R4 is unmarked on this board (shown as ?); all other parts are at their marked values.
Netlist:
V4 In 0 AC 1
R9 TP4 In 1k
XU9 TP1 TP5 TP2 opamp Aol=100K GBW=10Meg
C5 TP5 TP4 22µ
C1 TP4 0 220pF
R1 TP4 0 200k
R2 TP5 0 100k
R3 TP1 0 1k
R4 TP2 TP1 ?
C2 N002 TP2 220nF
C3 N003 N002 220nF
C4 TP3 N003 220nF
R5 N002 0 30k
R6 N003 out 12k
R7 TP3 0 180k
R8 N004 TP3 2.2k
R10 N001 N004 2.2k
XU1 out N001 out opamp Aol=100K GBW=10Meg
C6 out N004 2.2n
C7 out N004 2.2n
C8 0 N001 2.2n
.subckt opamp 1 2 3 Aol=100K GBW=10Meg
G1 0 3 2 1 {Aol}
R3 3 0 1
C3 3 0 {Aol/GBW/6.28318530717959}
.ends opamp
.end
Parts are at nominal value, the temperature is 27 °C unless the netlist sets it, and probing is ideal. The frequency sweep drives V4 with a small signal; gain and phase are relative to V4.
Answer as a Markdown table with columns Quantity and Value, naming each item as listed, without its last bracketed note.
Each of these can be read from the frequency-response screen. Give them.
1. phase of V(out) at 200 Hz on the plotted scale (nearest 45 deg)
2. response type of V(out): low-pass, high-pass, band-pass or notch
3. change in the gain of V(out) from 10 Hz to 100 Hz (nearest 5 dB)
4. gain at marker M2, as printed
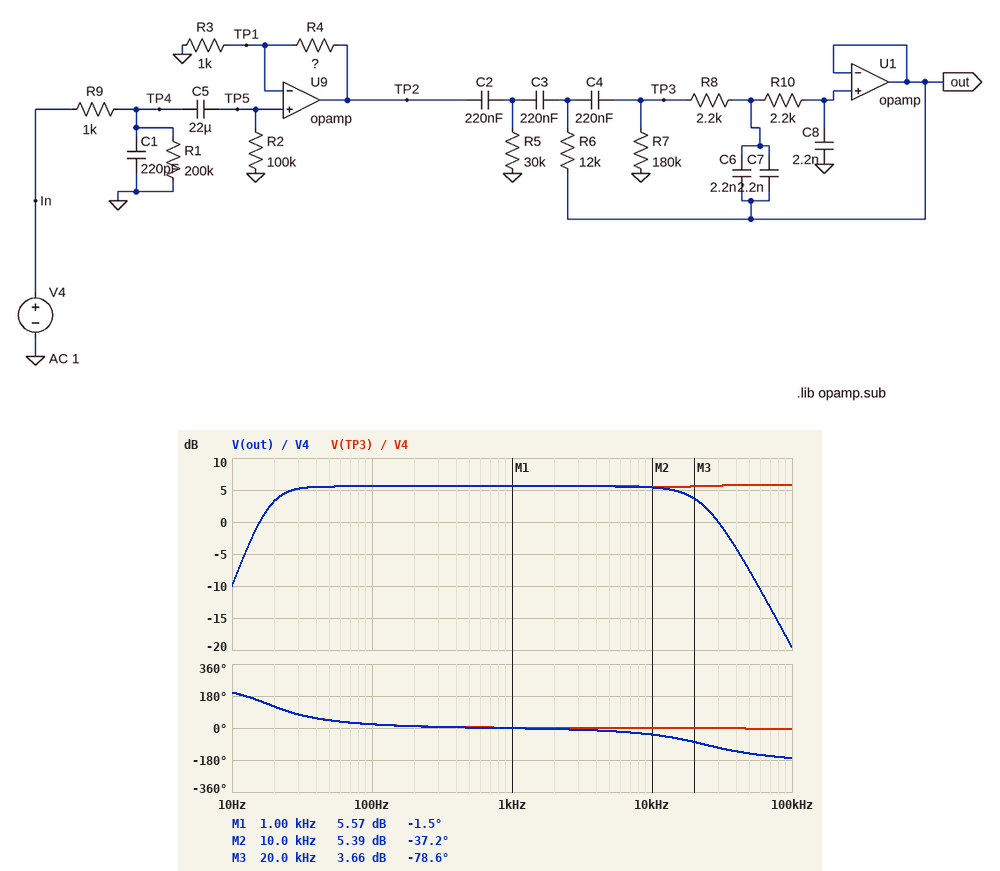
| Quantity | Value |
|---|---|
| phase of V(out) at 200 Hz on the plotted scale | 0 deg |
| response type of V(out): low-pass, high-pass, band-pass or notch | band-pass |
| change in the gain of V(out) from 10 Hz to 100 Hz | 15 dB |
| gain at marker M2, as printed | 5.39 dB |
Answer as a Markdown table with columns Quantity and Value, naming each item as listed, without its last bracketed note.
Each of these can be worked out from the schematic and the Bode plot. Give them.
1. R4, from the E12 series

| Quantity | Value |
|---|---|
| R4, from the E12 series | 1 kΩ |
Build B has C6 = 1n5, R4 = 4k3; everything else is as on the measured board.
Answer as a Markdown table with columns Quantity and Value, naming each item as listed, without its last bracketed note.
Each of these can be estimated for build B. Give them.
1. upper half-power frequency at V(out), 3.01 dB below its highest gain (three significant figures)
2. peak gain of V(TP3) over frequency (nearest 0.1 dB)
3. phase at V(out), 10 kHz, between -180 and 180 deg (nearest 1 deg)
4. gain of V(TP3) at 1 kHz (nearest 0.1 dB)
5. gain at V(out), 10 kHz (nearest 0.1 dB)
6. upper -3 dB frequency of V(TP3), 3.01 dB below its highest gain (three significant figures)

| Quantity | Value |
|---|---|
| upper half-power frequency at V(out), 3.01 dB below its highest gain | 23.2 kHz |
| peak gain of V(TP3) over frequency | 14.3 dB |
| phase at V(out), 10 kHz, between -180 and 180 deg | -36 deg |
| gain of V(TP3) at 1 kHz | 14.0 dB |
| gain at V(out), 10 kHz | 13.7 dB |
| upper -3 dB frequency of V(TP3), 3.01 dB below its highest gain | 663 kHz |
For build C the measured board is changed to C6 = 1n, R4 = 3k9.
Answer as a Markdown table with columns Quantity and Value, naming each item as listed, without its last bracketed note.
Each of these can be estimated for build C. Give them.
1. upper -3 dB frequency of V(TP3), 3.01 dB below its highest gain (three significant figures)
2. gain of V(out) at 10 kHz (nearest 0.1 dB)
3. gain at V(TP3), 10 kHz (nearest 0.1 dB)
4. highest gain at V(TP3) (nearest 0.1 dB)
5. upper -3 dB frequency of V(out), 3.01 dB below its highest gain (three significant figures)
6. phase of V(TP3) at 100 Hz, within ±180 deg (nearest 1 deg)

| Quantity | Value |
|---|---|
| upper -3 dB frequency of V(TP3), 3.01 dB below its highest gain | 673 kHz |
| gain of V(out) at 10 kHz | 12.9 dB |
| gain at V(TP3), 10 kHz | 13.4 dB |
| highest gain at V(TP3) | 13.6 dB |
| upper -3 dB frequency of V(out), 3.01 dB below its highest gain | 22.9 kHz |
| phase of V(TP3) at 100 Hz, within ±180 deg | 21 deg |
